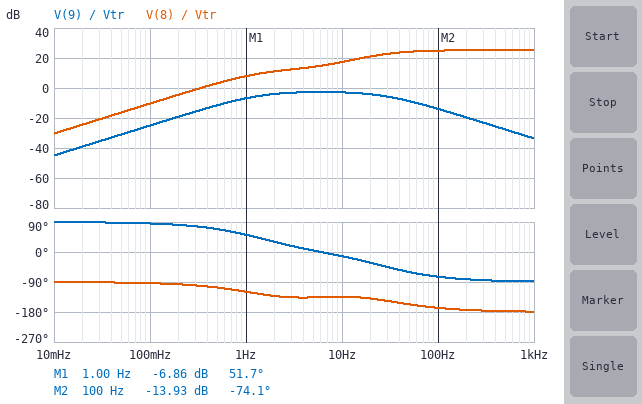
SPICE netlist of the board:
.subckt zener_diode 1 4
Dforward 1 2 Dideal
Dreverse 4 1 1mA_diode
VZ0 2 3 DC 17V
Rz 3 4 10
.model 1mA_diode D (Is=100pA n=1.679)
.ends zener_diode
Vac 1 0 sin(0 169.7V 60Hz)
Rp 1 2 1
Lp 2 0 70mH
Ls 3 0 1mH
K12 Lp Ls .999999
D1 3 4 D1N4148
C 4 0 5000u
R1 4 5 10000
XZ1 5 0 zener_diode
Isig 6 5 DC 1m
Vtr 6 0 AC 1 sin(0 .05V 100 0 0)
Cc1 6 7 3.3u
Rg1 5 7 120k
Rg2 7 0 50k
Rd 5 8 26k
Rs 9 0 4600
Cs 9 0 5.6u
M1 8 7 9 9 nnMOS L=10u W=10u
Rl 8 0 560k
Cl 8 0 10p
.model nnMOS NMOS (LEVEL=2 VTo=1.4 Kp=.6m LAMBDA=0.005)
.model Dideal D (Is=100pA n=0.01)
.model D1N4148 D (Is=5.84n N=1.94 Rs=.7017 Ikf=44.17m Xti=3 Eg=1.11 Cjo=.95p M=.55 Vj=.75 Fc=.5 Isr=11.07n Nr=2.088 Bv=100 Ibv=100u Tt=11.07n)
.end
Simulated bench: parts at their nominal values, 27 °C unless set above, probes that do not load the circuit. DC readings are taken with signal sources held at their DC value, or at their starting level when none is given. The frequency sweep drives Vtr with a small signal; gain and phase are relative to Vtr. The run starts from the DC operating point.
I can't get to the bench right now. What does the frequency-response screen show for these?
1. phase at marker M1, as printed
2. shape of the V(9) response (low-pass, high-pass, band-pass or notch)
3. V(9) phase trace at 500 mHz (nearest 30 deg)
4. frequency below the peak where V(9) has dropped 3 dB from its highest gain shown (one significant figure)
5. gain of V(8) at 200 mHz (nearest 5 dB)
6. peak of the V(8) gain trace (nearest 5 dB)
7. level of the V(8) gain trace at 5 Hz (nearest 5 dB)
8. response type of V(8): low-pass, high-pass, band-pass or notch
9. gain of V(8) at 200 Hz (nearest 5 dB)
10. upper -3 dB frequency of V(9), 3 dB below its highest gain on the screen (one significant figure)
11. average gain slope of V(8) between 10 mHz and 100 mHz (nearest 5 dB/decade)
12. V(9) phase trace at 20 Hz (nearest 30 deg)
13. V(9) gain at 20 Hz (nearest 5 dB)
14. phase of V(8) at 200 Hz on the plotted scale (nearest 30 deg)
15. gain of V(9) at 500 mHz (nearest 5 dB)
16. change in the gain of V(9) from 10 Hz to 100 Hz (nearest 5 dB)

51.7 deg
band-pass
60 deg
1 Hz
-5 dB
25 dB
15 dB
high-pass
25 dB
30 Hz
20 dB/decade
-30 deg
-5 dB
-180 deg
-10 dB
-10 dB
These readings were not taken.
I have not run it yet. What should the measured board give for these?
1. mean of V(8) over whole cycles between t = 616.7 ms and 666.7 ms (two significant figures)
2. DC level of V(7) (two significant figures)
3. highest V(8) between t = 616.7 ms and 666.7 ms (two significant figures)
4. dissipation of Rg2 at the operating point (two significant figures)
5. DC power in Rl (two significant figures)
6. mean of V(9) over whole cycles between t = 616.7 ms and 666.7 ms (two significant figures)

3.8 V
5.0 V
4.5 V
500 µW
25 µW
2.3 V
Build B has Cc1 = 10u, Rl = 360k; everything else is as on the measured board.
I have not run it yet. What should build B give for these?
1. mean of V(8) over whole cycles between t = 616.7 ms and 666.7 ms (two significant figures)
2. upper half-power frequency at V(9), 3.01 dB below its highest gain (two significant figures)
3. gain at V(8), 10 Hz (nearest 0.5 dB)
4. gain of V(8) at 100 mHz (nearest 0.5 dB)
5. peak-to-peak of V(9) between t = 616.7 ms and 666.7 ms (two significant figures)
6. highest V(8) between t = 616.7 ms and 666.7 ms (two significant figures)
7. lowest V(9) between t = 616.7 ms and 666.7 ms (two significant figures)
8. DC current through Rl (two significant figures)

3.7 V
28 Hz
17.0 dB
-1.0 dB
13 mV
4.4 V
2.3 V
10 µA
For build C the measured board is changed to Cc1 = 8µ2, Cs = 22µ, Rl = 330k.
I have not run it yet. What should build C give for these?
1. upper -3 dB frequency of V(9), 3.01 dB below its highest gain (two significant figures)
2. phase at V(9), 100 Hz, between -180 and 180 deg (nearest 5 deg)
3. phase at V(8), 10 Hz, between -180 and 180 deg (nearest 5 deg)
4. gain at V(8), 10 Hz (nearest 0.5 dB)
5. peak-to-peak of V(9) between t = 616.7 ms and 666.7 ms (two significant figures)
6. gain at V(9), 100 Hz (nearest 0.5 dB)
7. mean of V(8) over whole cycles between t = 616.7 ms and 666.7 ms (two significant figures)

7.9 Hz
-85 deg
-150 deg
23.5 dB
3.3 mV
-25.5 dB
3.7 V
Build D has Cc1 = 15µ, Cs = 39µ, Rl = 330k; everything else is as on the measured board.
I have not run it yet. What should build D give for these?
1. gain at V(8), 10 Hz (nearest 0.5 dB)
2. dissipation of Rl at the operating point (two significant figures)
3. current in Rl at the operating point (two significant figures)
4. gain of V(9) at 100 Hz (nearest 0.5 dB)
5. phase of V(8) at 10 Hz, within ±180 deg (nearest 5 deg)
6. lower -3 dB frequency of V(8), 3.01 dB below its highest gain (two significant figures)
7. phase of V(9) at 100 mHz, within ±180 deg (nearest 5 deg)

24.5 dB
40 µW
11 µA
-30.5 dB
-160 deg
3.7 Hz
70 deg
